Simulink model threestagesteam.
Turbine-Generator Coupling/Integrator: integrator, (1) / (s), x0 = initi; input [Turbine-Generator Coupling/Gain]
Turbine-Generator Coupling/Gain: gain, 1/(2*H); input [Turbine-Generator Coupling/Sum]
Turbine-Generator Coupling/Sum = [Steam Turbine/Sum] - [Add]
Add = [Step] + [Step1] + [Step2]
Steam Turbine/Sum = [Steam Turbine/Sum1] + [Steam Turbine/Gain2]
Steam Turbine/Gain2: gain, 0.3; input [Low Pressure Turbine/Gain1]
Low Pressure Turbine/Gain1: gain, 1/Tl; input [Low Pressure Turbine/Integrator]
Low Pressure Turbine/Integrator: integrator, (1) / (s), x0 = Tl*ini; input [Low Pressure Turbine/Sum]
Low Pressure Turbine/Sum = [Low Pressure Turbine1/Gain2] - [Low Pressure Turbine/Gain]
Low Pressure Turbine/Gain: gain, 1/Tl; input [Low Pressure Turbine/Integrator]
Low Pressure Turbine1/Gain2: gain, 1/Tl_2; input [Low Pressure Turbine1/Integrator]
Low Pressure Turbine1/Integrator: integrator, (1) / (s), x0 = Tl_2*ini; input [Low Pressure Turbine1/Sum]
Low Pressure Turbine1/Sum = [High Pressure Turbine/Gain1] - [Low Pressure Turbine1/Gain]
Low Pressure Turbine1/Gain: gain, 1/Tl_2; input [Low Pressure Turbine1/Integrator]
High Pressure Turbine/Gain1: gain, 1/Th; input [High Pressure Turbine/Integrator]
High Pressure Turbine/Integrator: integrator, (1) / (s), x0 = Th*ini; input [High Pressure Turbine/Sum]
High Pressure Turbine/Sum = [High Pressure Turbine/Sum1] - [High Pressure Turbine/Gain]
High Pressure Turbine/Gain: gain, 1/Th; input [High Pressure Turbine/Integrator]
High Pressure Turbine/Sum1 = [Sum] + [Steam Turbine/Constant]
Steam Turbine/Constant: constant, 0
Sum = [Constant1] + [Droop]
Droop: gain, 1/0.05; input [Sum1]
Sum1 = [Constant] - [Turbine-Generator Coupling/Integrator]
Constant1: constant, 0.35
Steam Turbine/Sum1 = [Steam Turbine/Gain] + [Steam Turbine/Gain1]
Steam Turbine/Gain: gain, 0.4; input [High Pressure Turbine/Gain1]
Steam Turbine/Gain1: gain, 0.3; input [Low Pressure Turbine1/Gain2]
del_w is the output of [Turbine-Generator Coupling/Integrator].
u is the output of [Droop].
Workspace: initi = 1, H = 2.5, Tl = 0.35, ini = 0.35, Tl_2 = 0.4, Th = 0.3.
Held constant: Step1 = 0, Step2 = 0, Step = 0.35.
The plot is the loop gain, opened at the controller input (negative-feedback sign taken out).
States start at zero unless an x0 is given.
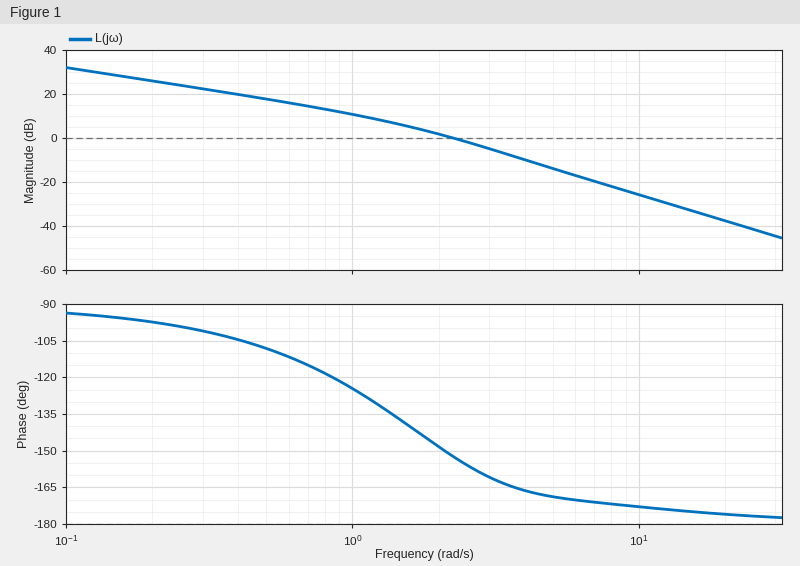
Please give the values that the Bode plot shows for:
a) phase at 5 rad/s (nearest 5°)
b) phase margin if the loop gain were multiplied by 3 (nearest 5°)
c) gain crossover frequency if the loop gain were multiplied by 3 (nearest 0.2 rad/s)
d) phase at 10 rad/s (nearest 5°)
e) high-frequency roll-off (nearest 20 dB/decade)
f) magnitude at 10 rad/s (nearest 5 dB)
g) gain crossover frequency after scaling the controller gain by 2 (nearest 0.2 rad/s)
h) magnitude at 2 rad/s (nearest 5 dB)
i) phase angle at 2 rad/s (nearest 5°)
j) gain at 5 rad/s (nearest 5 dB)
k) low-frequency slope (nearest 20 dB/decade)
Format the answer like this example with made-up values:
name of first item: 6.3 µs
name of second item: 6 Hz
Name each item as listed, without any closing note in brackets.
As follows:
phase at 5 rad/s: -170°
phase margin if the loop gain were multiplied by 3: 15°
gain crossover frequency if the loop gain were multiplied by 3: 4.0 rad/s
phase at 10 rad/s: -175°
high-frequency roll-off: -40 dB/decade
magnitude at 10 rad/s: -25 dB
gain crossover frequency after scaling the controller gain by 2: 3.2 rad/s
magnitude at 2 rad/s: 0 dB
phase angle at 2 rad/s: -150°
gain at 5 rad/s: -15 dB
low-frequency slope: -20 dB/decade
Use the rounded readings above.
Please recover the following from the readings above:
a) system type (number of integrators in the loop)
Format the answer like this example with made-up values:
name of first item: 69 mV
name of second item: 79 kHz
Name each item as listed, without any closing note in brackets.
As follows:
system type: 1
